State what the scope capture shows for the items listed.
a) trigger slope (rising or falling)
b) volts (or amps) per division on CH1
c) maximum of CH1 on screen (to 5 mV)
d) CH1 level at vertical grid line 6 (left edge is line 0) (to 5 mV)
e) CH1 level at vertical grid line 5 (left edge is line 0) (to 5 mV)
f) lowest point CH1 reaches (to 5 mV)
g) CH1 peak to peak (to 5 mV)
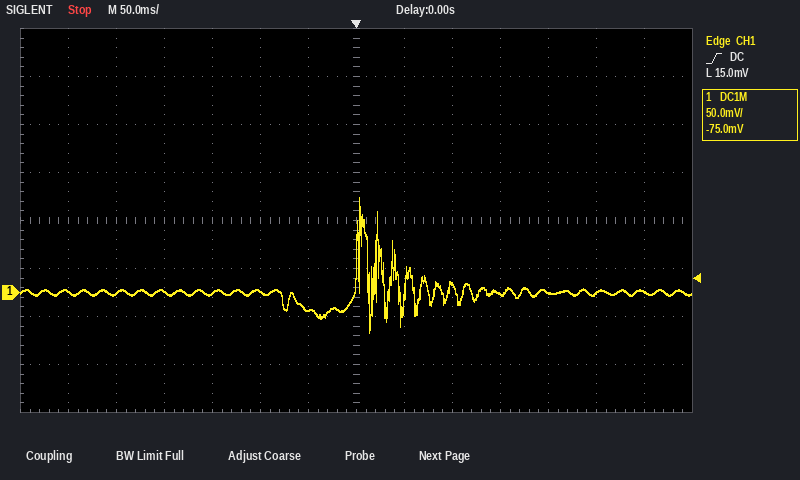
rising
50 mV
100 mV
-20 mV
0 mV
-40 mV
140 mV
